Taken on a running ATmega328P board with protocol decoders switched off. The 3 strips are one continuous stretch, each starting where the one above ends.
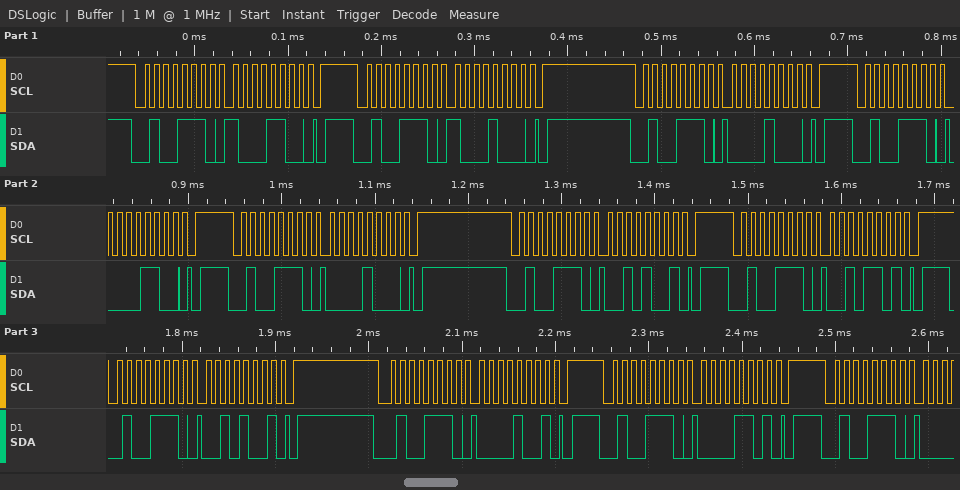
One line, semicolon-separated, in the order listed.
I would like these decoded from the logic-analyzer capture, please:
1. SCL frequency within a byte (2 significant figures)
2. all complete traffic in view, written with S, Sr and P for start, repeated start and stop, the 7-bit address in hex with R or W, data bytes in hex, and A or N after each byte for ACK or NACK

100 kHz; S 27W A 8C A P S 27W A 88 A P S 27W A 08 A P S 27W A 0C A P S 27W A 08 A P S 27W A 29 A P S 27W A 2D A P S 27W A 29 A P S 27W A 09 A P S 27W A 0D A P S 27W A
